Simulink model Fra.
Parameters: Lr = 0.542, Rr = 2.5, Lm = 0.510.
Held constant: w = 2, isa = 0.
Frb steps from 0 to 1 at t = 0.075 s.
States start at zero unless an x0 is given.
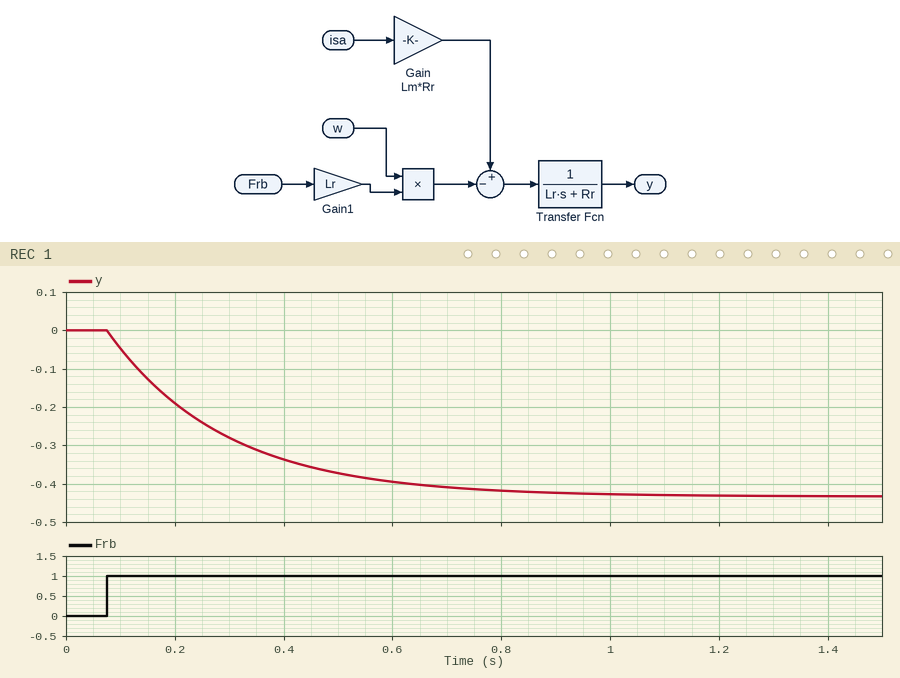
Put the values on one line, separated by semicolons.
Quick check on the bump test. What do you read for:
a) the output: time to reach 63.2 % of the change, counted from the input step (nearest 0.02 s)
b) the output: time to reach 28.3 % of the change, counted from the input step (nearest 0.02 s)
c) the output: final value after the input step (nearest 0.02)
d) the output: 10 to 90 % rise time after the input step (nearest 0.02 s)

0.22 s; 0.08 s; -0.44; 0.48 s
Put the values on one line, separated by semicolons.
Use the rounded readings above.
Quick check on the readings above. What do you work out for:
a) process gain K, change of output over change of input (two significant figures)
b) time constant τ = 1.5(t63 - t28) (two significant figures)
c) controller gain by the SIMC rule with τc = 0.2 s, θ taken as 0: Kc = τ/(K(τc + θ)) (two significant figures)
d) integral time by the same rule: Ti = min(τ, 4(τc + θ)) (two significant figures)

-0.44; 0.21 s; -2.4; 0.21 s
